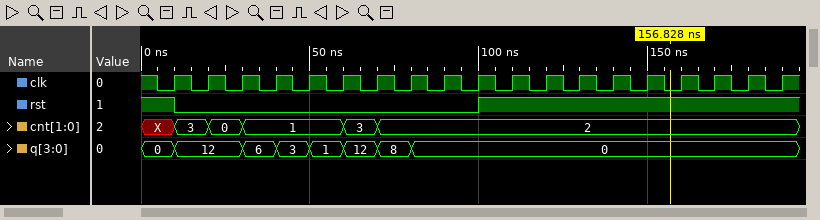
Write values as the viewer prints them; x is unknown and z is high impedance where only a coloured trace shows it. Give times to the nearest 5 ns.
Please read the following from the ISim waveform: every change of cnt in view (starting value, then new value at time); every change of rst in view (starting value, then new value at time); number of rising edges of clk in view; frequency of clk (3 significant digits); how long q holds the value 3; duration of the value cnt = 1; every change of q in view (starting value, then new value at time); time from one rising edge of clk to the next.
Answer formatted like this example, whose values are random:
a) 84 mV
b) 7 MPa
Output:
a) X, 3 at 10 ns, 0 at 20 ns, 1 at 30 ns, 3 at 60 ns, 2 at 70 ns
b) 1, 0 at 10 ns, 1 at 100 ns
c) 19
d) 100 MHz
e) 10 ns
f) 30 ns
g) 0, 12 at 10 ns, 6 at 30 ns, 3 at 40 ns, 1 at 50 ns, 12 at 60 ns, 8 at 70 ns, 0 at 80 ns
h) 10 ns
